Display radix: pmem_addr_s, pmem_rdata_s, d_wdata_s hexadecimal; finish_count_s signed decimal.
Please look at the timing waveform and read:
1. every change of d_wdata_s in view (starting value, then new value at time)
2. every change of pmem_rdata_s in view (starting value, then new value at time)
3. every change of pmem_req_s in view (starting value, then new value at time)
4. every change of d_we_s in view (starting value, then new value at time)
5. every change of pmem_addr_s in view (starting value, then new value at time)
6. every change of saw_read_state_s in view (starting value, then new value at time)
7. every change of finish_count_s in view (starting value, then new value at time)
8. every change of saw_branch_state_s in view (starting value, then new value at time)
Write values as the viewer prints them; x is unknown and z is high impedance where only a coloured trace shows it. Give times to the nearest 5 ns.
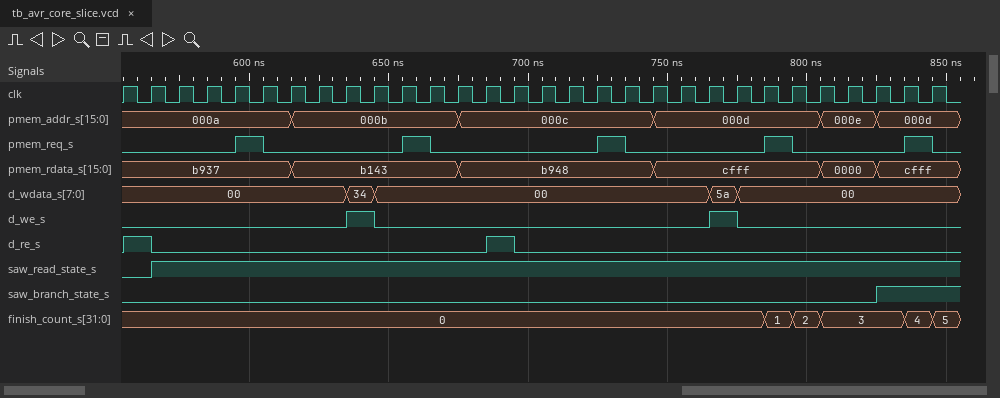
00, 34 at 635 ns, 00 at 645 ns, 5a at 765 ns, 00 at 775 ns
b937, b143 at 615 ns, b948 at 675 ns, cfff at 745 ns, 0000 at 805 ns, cfff at 825 ns
0, 1 at 595 ns, 0 at 605 ns, 1 at 655 ns, 0 at 665 ns, 1 at 725 ns, 0 at 735 ns, 1 at 785 ns, 0 at 795 ns, 1 at 835 ns, 0 at 845 ns
0, 1 at 635 ns, 0 at 645 ns, 1 at 765 ns, 0 at 775 ns
000a, 000b at 615 ns, 000c at 675 ns, 000d at 745 ns, 000e at 805 ns, 000d at 825 ns
0, 1 at 565 ns
0, 1 at 785 ns, 2 at 795 ns, 3 at 805 ns, 4 at 835 ns, 5 at 845 ns
0, 1 at 825 ns
